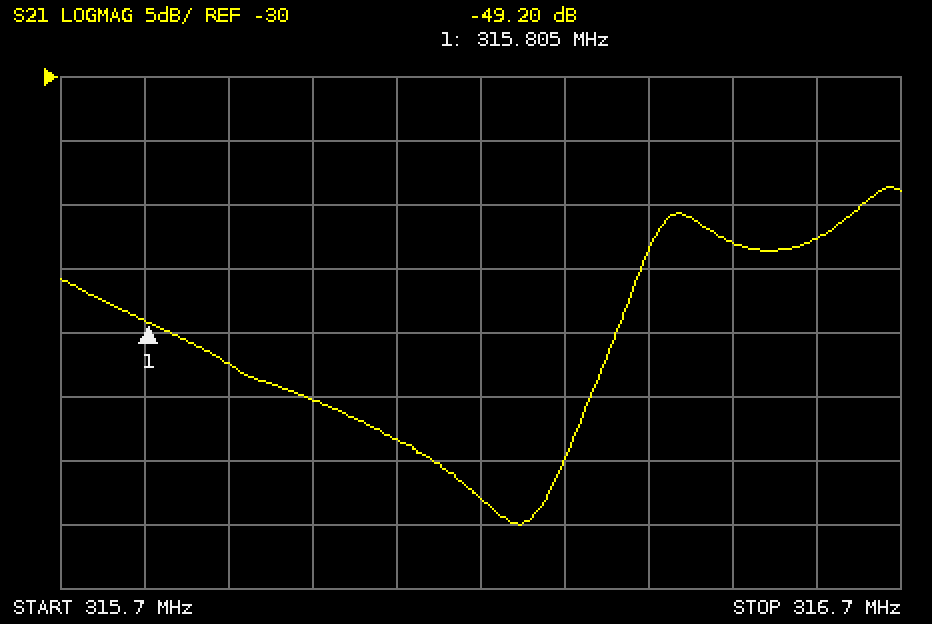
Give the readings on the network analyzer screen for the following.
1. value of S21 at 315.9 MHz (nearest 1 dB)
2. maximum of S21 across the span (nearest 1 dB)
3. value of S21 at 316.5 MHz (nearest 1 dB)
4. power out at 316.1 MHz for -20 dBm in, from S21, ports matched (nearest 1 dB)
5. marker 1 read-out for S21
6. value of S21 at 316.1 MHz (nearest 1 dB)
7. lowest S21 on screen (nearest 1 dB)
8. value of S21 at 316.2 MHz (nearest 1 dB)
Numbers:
-52 dB
-39 dB
-43 dB
-78 dBm
-49.20 dB
-58 dB
-65 dB
-63 dB
